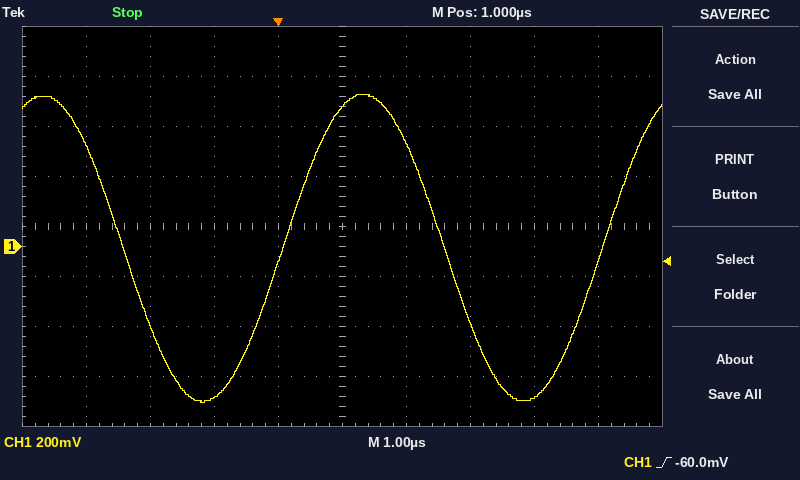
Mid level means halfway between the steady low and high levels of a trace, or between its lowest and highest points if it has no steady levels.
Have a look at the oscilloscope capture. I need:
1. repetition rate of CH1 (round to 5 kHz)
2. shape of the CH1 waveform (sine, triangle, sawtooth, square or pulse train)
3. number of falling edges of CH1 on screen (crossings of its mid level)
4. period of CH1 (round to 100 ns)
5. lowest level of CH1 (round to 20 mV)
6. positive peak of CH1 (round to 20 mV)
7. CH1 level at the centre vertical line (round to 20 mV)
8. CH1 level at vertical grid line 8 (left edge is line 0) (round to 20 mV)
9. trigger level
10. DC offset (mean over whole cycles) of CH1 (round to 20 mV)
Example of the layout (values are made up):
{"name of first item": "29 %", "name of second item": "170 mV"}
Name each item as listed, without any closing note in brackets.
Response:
{"repetition rate of CH1": "200 kHz", "shape of the CH1 waveform": "sine", "number of falling edges of CH1 on screen": "2", "period of CH1": "5.0 µs", "lowest level of CH1": "-620 mV", "positive peak of CH1": "600 mV", "CH1 level at the centre vertical line": "560 mV", "CH1 level at vertical grid line 8 (left edge is line 0)": "-600 mV", "trigger level": "-60.0 mV", "DC offset (mean over whole cycles) of CH1": "0 mV"}
